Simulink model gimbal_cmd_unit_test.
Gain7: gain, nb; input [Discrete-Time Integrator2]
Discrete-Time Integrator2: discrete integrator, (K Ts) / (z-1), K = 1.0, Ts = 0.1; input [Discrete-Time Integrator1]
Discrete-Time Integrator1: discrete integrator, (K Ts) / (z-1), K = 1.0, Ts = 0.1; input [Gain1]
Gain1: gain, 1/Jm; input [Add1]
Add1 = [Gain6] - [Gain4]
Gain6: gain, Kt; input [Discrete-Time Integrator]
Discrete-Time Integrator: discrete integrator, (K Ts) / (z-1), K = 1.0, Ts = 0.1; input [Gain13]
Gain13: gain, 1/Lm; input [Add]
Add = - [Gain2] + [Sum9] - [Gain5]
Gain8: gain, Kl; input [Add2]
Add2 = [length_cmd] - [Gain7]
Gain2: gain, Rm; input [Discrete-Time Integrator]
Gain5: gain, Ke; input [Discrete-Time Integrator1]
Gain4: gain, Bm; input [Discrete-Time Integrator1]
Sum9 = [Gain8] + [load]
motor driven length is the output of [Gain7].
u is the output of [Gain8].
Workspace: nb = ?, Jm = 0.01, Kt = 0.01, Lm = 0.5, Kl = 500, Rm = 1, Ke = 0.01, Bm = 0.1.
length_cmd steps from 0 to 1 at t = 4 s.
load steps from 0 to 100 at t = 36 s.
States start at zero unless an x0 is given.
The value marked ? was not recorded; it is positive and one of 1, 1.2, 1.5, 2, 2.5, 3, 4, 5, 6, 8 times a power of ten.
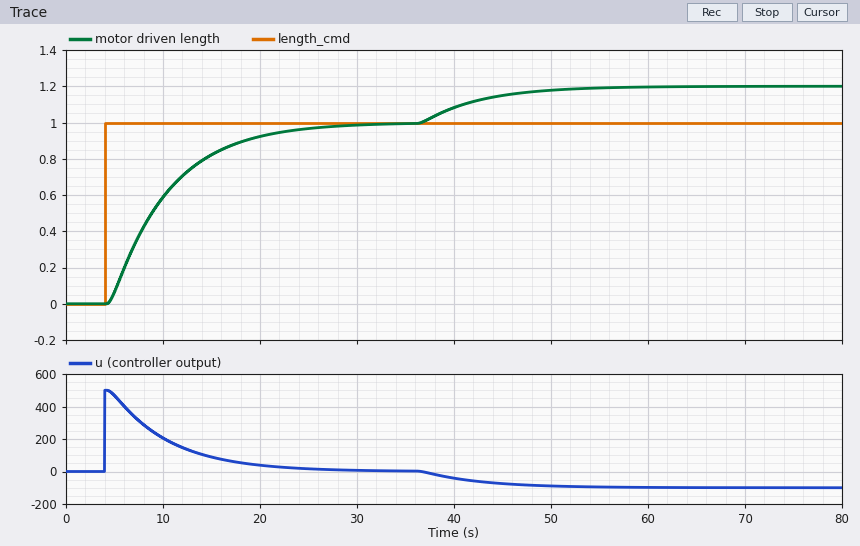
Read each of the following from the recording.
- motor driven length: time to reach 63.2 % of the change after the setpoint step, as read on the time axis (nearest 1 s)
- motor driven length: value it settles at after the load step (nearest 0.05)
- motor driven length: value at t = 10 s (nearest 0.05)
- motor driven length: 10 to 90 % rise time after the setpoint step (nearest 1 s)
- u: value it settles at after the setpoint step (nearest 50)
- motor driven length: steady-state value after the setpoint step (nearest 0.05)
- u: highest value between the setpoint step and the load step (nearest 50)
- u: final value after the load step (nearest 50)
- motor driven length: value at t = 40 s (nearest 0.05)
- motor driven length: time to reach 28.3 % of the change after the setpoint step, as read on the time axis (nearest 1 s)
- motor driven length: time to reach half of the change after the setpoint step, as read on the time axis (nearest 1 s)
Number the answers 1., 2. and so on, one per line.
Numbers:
1. 11 s
2. 1.20
3. 0.60
4. 13 s
5. 0
6. 1.00
7. 500
8. -100
9. 1.10
10. 7 s
11. 9 s
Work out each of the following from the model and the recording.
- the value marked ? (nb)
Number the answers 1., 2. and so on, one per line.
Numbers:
1. 0.003
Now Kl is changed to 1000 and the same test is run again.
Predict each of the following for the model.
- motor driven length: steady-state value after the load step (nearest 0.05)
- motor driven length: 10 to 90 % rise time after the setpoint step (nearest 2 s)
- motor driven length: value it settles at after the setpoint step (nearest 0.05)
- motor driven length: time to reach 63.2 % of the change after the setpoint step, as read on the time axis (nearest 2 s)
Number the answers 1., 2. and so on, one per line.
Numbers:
1. 1.10
2. 6 s
3. 1.00
4. 8 s
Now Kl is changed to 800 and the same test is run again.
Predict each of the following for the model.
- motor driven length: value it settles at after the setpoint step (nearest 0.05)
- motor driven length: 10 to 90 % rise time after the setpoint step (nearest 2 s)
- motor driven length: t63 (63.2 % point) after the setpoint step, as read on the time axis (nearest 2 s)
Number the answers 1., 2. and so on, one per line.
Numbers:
1. 1.00
2. 8 s
3. 8 s
